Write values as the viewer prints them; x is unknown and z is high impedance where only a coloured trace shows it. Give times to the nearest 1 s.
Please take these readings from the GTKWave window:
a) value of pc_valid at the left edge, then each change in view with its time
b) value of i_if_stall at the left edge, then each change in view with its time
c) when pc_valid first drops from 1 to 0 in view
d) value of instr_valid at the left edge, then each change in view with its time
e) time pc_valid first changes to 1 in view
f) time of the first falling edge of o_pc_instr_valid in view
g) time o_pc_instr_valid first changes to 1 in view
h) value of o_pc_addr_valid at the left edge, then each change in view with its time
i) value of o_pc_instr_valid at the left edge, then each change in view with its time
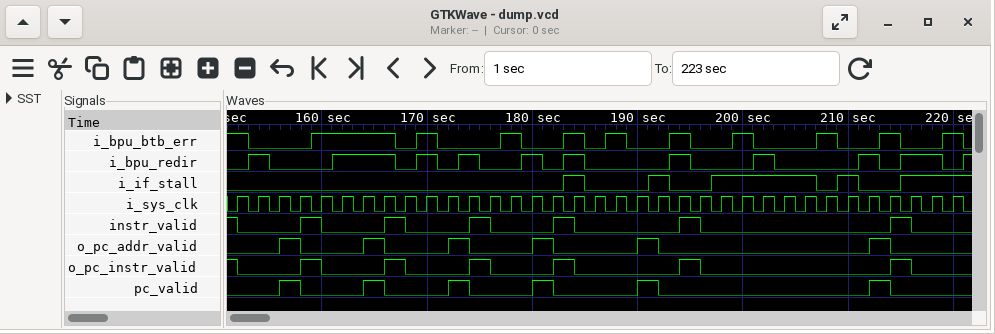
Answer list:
0, 1 at 156 s, 0 at 158 s, 1 at 164 s, 0 at 166 s, 1 at 172 s, 0 at 174 s, 1 at 180 s, 0 at 182 s, 1 at 190 s, 0 at 192 s, 1 at 212 s, 0 at 214 s
0, 1 at 183 s, 0 at 185 s, 1 at 191 s, 0 at 193 s, 1 at 197 s, 0 at 207 s, 1 at 209 s, 0 at 211 s, 1 at 215 s
158 s
1, 0 at 152 s, 1 at 158 s, 0 at 160 s, 1 at 166 s, 0 at 168 s, 1 at 174 s, 0 at 176 s, 1 at 182 s, 0 at 184 s, 1 at 194 s, 0 at 196 s, 1 at 214 s, 0 at 216 s
156 s
152 s
158 s
0, 1 at 156 s, 0 at 158 s, 1 at 164 s, 0 at 166 s, 1 at 172 s, 0 at 174 s, 1 at 180 s, 0 at 182 s, 1 at 190 s, 0 at 192 s, 1 at 212 s, 0 at 214 s
1, 0 at 152 s, 1 at 158 s, 0 at 160 s, 1 at 166 s, 0 at 168 s, 1 at 174 s, 0 at 176 s, 1 at 182 s, 0 at 184 s, 1 at 194 s, 0 at 196 s, 1 at 214 s, 0 at 216 s
